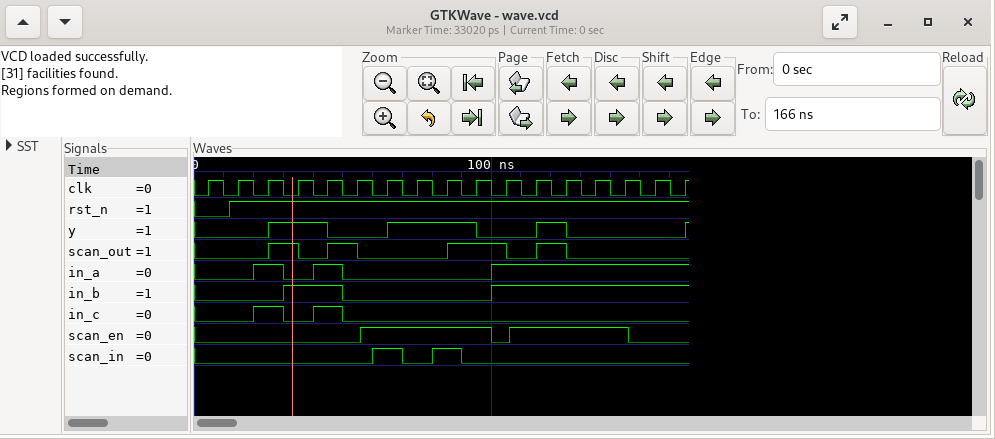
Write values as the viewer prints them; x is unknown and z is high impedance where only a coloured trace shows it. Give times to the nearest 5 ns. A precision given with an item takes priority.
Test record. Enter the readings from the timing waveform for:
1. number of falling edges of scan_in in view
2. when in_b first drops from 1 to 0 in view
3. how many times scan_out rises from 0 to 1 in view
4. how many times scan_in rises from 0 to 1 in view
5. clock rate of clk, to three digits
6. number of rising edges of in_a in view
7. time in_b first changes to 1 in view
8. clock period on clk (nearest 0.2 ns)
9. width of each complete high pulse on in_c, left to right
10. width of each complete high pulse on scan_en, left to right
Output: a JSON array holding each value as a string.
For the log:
["2", "50 ns", "4", "2", "100 MHz", "3", "30 ns", "10 ns", "10 ns, 10 ns", "45 ns, 40 ns"]
